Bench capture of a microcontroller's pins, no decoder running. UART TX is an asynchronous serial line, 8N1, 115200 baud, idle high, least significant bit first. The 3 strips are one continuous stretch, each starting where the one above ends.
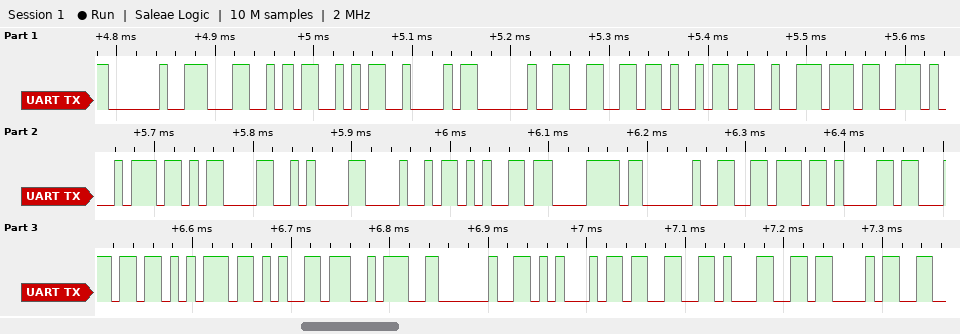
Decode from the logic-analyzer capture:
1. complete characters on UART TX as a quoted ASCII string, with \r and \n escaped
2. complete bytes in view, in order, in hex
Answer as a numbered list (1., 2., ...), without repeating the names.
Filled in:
1. " LSB first\r\nHex value: E31C"
2. 20 4C 53 42 20 66 69 72 73 74 0D 0A 48 65 78 20 76 61 6C 75 65 3A 20 45 33 31 43
